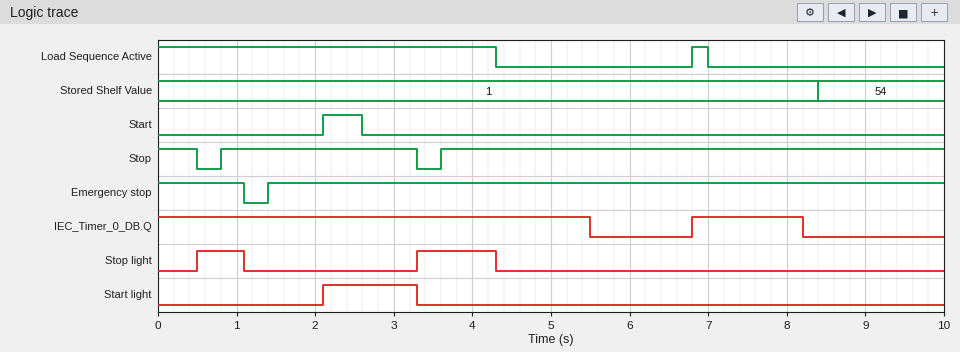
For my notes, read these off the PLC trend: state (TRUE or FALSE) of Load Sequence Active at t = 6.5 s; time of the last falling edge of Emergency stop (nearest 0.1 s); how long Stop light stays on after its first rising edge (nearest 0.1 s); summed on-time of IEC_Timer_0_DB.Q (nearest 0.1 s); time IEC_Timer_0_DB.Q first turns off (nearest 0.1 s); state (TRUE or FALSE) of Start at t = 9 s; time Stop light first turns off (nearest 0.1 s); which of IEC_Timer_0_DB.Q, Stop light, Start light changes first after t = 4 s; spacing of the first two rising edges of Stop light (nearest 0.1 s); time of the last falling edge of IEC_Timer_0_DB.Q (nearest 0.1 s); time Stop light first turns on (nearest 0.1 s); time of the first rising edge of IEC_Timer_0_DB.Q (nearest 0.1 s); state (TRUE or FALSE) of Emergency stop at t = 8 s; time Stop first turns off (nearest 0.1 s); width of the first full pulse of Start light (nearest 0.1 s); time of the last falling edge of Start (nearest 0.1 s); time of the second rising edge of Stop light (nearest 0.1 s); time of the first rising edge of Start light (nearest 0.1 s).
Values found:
FALSE
1.1 s
0.6 s
6.9 s
5.5 s
FALSE
1.1 s
Stop light
2.8 s
8.2 s
0.5 s
6.8 s
TRUE
0.5 s
1.2 s
2.6 s
3.3 s
2.1 s
